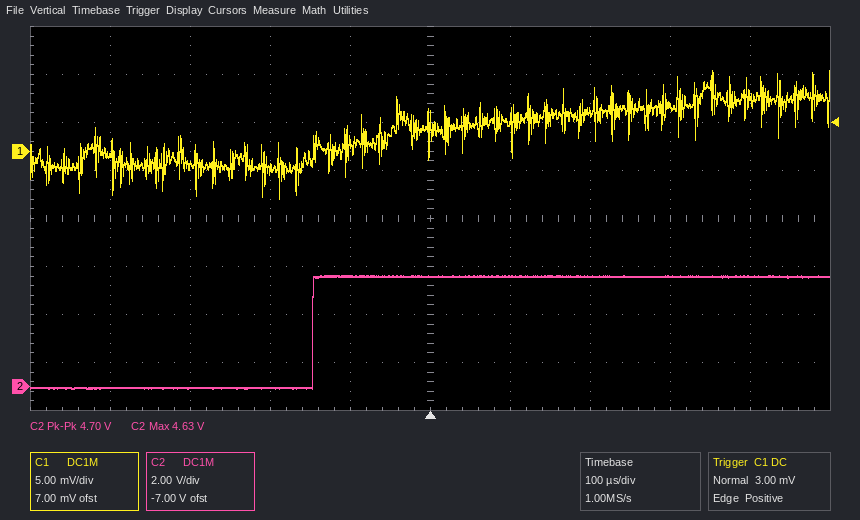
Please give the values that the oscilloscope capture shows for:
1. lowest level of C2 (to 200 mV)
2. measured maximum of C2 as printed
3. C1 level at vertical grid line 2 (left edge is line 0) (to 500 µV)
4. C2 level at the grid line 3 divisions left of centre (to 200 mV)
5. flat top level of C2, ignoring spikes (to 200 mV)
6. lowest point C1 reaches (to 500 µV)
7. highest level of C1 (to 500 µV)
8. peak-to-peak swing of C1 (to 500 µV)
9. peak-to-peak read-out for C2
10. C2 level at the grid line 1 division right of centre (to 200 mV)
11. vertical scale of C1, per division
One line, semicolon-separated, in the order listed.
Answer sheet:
0.0 V; 4.63 V; -1.5 mV; 0.0 V; 4.6 V; -5.0 mV; 8.5 mV; 13.5 mV; 4.70 V; 4.6 V; 5 mV
